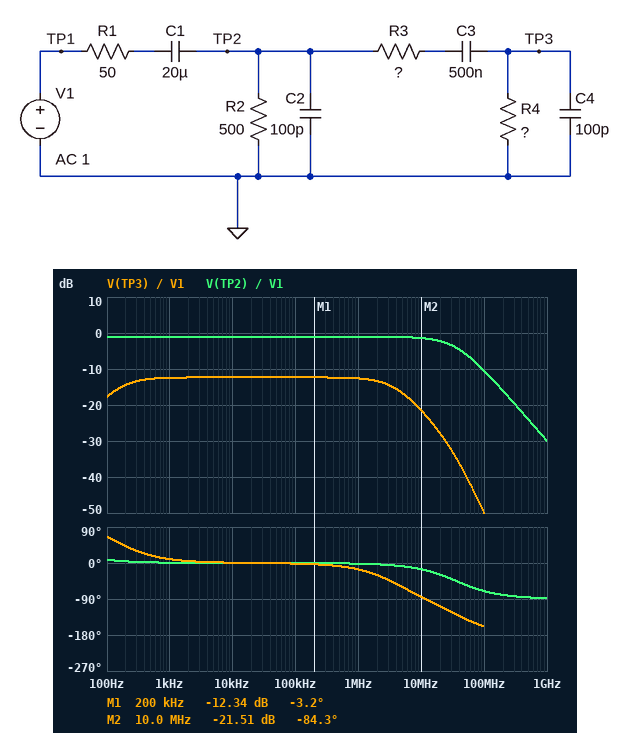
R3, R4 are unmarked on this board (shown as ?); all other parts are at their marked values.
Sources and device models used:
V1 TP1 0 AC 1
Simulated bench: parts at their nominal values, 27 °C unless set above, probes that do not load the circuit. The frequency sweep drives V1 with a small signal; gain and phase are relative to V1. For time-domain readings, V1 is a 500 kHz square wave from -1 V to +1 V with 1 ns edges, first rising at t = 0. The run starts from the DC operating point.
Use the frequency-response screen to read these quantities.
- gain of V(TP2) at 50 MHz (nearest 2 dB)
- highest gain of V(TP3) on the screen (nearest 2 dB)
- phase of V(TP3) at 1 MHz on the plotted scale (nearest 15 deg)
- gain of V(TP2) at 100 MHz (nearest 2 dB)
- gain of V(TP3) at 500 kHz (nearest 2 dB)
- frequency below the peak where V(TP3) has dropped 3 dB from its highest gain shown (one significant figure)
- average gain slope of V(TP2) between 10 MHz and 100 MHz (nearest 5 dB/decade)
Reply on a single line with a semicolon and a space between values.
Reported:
-6 dB; -12 dB; -15 deg; -10 dB; -12 dB; 200 Hz; -10 dB/decade
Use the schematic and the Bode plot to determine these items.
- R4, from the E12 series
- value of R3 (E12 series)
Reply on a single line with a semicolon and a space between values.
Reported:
560 Ω; 1.5 kΩ
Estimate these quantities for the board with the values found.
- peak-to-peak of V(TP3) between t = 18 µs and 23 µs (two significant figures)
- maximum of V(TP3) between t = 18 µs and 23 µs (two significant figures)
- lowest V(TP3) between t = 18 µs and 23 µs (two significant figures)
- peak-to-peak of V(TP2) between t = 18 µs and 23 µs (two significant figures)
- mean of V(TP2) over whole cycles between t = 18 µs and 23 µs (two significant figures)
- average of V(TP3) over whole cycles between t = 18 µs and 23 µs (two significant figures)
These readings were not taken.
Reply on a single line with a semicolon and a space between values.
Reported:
480 mV; 480 mV; -5.6 mV; 1.8 V; 890 mV; 240 mV
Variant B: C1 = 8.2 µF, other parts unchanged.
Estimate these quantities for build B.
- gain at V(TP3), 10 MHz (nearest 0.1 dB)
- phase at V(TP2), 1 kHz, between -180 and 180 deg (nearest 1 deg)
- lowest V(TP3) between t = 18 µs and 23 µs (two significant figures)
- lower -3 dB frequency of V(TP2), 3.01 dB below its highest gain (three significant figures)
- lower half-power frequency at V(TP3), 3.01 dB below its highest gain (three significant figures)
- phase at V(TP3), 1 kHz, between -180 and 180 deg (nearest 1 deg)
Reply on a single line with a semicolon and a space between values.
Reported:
-21.5 dB; 2 deg; -6.4 mV; 35.9 Hz; 167 Hz; 11 deg
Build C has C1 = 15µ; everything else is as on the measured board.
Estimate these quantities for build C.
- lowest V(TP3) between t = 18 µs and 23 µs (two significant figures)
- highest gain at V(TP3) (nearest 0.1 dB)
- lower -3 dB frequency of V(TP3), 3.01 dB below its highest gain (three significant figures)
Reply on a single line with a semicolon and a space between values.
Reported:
-5.8 mV; -12.3 dB; 158 Hz
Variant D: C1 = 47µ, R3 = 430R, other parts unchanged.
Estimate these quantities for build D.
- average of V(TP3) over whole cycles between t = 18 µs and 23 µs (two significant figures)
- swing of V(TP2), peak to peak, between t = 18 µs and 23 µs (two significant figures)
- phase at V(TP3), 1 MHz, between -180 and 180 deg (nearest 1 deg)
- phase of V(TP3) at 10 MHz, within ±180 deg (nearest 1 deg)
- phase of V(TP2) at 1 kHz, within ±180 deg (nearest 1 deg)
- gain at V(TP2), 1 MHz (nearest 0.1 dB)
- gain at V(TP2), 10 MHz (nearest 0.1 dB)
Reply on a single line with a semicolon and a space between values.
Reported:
470 mV; 1.7 V; -11 deg; -73 deg; 0 deg; -1.2 dB; -1.9 dB
